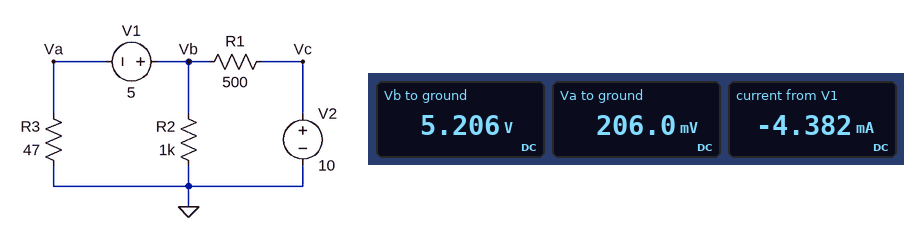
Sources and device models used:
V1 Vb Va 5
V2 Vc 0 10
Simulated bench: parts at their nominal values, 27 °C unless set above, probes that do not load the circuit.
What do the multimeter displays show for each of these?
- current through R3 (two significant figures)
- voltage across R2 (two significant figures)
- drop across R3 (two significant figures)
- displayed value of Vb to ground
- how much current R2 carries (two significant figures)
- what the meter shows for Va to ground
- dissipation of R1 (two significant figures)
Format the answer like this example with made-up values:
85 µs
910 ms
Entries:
4.4 mA
5.2 V
210 mV
5.206 V
5.2 mA
206.0 mV
46 mW
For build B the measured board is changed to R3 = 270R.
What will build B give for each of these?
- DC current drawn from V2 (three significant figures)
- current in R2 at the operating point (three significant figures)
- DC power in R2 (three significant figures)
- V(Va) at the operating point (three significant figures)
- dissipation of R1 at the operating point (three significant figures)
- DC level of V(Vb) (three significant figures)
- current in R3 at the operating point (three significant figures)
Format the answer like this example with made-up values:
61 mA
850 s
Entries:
8.51 mA
5.75 mA
33.0 mW
746 mV
36.2 mW
5.75 V
2.76 mA
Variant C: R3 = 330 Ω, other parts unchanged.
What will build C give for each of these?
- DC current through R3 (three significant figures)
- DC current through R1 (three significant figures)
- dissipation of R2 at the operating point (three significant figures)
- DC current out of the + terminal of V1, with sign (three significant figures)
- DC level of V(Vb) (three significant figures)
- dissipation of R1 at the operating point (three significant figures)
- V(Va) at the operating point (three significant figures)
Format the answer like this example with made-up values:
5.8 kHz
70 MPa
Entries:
2.51 mA
8.34 mA
34.0 mW
-2.51 mA
5.83 V
34.8 mW
829 mV
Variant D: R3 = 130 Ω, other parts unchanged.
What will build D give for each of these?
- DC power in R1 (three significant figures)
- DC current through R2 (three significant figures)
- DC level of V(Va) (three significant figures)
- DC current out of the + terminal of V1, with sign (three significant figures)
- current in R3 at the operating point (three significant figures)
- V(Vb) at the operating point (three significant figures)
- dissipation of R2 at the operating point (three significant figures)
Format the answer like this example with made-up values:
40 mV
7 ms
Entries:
41.1 mW
5.47 mA
468 mV
-3.60 mA
3.60 mA
5.47 V
29.9 mW
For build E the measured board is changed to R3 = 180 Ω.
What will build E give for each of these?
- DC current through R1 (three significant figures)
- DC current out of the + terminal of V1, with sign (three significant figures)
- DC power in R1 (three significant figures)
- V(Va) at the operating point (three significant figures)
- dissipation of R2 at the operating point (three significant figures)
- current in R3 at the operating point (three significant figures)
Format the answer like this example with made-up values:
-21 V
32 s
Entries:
8.83 mA
-3.25 mA
39.0 mW
584 mV
31.2 mW
3.25 mA
